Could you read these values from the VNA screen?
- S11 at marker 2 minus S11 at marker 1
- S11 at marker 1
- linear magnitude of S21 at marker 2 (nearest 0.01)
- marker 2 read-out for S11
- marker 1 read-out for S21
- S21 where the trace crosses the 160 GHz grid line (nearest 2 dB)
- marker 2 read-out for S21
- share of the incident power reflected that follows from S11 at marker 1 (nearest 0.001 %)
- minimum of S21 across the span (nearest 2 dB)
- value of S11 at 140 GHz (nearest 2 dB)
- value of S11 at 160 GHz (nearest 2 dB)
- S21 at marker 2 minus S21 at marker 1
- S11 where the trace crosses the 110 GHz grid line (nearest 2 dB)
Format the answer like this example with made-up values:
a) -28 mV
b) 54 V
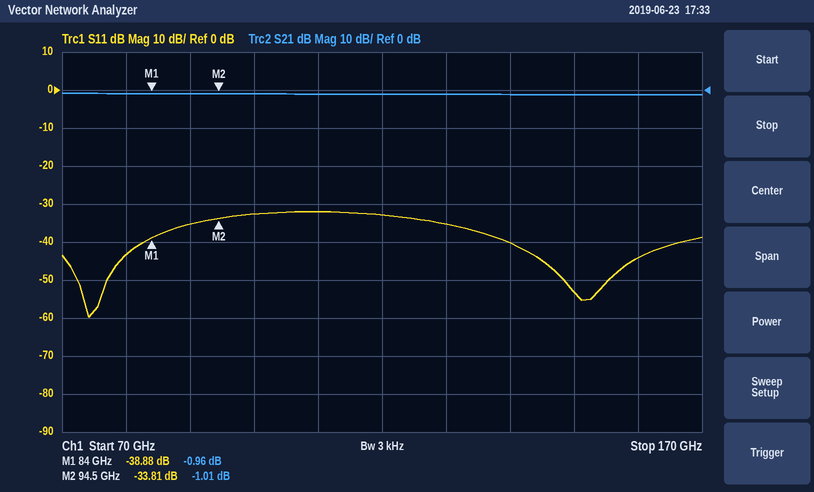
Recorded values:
a) 5.07 dB
b) -38.88 dB
c) 0.89
d) -33.81 dB
e) -0.96 dB
f) -2 dB
g) -1.01 dB
h) 0.013 %
i) -2 dB
j) -40 dB
k) -44 dB
l) -0.05 dB
m) -32 dB
